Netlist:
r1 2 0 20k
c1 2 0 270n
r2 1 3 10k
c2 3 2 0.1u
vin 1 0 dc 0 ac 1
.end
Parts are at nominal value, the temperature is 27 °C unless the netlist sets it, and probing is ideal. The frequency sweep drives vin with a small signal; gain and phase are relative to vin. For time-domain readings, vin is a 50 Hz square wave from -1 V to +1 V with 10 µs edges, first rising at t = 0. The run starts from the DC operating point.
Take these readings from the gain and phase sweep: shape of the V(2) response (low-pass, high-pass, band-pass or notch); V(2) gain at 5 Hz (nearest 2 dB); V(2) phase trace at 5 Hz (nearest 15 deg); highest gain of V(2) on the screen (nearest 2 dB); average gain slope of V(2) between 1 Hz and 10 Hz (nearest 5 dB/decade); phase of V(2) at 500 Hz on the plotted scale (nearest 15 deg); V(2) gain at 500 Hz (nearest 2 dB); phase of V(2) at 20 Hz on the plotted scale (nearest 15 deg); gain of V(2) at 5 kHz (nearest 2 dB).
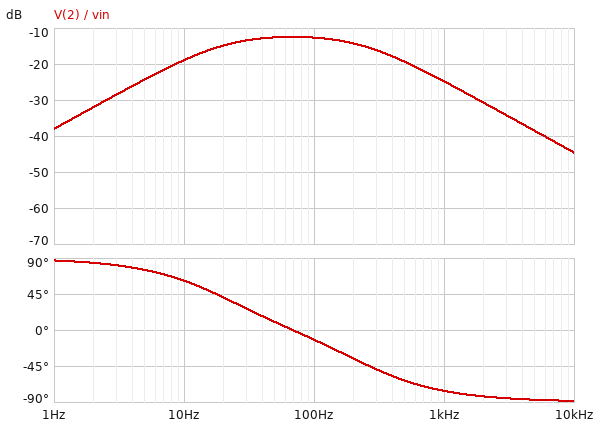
band-pass
-24 dB
75 deg
-12 dB
20 dB/decade
-60 deg
-20 dB
45 deg
-38 dB
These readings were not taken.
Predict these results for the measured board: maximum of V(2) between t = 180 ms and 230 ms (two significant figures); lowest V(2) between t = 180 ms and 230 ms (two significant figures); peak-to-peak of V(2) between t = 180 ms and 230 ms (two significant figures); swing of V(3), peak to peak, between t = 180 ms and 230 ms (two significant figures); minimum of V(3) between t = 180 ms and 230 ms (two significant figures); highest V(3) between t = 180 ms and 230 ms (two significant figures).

310 mV
-310 mV
630 mV
2.0 V
-980 mV
980 mV
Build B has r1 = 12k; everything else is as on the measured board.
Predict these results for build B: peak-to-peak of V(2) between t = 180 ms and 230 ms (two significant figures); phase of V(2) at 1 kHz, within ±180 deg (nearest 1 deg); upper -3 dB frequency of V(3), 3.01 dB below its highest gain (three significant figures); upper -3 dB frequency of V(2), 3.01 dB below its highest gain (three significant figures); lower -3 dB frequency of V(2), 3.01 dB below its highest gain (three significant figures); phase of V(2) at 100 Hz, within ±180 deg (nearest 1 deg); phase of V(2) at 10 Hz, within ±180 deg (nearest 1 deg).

640 mV
-75 deg
202 Hz
294 Hz
26.6 Hz
-5 deg
71 deg
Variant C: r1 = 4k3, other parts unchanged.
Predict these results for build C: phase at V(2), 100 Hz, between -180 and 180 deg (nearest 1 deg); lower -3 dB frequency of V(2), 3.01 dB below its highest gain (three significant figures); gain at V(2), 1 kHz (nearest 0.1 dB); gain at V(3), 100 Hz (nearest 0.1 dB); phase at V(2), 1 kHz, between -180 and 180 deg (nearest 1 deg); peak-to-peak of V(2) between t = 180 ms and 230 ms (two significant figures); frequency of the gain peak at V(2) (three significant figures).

18 deg
53.4 Hz
-24.9 dB
-1.7 dB
-70 deg
510 mV
148 Hz
